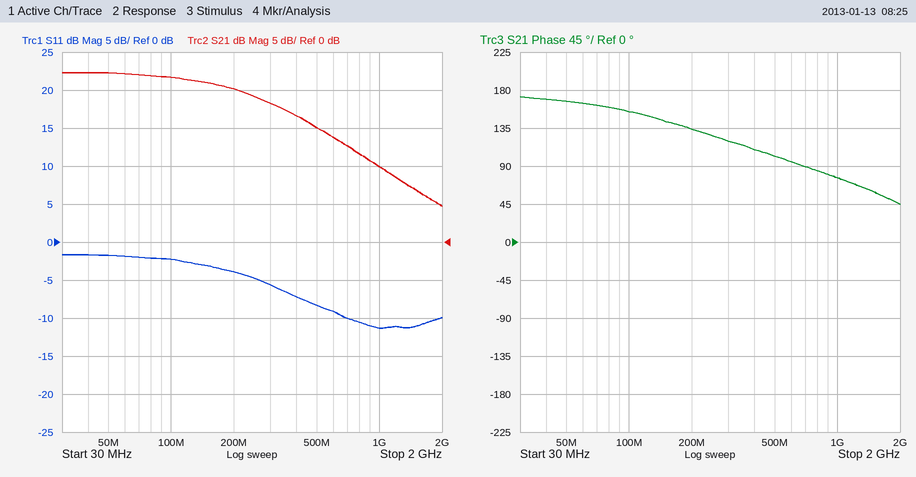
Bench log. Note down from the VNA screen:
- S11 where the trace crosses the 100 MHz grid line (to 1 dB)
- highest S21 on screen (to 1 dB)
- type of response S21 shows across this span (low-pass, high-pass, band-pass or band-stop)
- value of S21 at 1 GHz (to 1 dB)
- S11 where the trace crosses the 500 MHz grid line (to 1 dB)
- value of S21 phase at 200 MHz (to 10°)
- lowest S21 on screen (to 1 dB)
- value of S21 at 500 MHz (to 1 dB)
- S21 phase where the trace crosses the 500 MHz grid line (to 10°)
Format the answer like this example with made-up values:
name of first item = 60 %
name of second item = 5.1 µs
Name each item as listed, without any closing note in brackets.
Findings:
S11 where the trace crosses the 100 MHz grid line = -2 dB
highest S21 on screen = 22 dB
type of response S21 shows across this span = low-pass
value of S21 at 1 GHz = 10 dB
S11 where the trace crosses the 500 MHz grid line = -8 dB
value of S21 phase at 200 MHz = 130°
lowest S21 on screen = 5 dB
value of S21 at 500 MHz = 15 dB
S21 phase where the trace crosses the 500 MHz grid line = 100°
